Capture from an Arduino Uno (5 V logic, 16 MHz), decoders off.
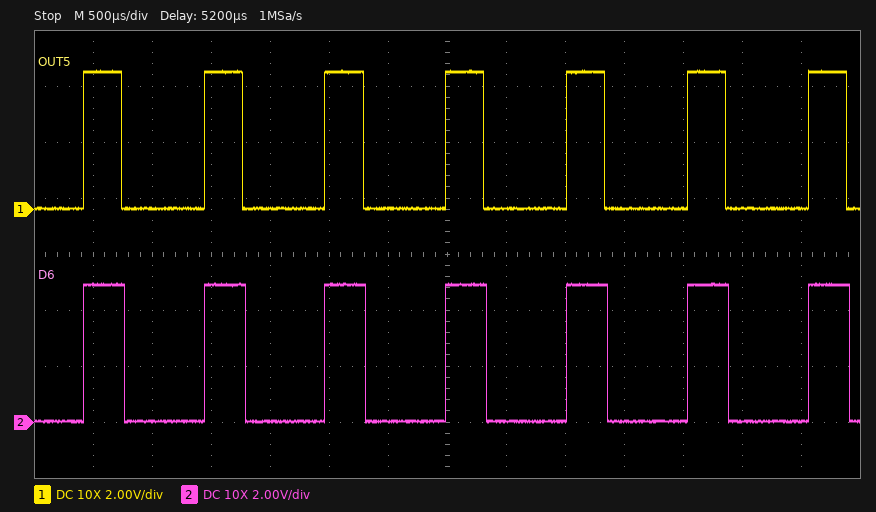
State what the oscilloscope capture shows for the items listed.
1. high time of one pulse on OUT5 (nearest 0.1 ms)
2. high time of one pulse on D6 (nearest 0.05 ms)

0.3 ms
0.35 ms
